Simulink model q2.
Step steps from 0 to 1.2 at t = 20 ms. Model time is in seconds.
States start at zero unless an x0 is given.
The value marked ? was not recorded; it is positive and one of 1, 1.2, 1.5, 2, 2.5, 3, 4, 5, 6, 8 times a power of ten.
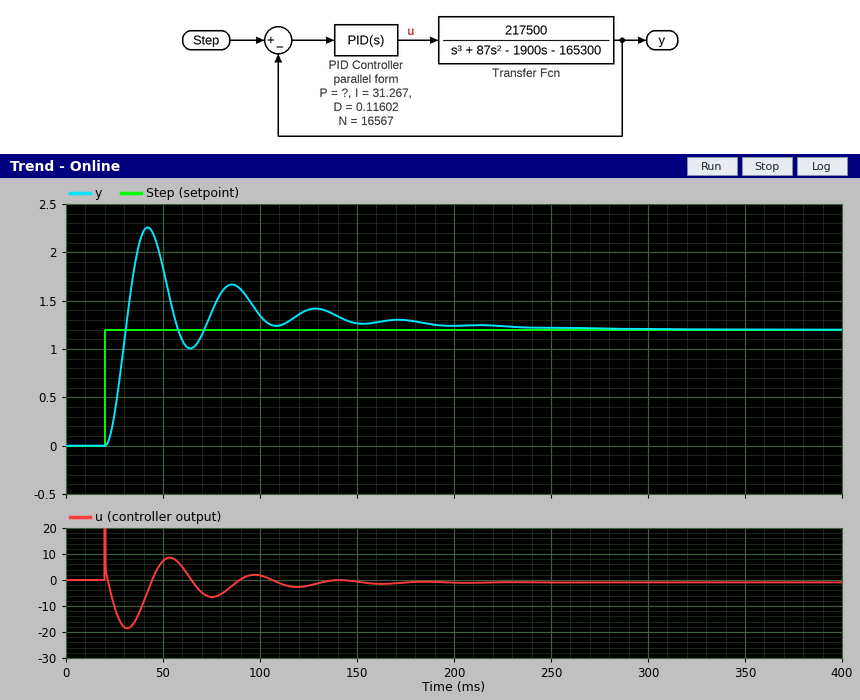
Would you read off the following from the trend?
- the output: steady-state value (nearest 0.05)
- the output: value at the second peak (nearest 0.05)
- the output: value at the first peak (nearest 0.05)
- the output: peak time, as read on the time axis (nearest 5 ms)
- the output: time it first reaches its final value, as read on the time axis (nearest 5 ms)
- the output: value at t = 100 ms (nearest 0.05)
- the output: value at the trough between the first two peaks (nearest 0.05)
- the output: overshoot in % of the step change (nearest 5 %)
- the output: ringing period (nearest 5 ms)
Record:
1.20
1.65
2.25
40 ms
30 ms
1.35
1.00
90 %
45 ms
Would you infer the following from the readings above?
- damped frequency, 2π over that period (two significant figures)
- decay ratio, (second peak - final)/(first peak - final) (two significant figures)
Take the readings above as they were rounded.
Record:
0.14 rad/ms
0.43
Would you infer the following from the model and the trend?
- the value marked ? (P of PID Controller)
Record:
4
